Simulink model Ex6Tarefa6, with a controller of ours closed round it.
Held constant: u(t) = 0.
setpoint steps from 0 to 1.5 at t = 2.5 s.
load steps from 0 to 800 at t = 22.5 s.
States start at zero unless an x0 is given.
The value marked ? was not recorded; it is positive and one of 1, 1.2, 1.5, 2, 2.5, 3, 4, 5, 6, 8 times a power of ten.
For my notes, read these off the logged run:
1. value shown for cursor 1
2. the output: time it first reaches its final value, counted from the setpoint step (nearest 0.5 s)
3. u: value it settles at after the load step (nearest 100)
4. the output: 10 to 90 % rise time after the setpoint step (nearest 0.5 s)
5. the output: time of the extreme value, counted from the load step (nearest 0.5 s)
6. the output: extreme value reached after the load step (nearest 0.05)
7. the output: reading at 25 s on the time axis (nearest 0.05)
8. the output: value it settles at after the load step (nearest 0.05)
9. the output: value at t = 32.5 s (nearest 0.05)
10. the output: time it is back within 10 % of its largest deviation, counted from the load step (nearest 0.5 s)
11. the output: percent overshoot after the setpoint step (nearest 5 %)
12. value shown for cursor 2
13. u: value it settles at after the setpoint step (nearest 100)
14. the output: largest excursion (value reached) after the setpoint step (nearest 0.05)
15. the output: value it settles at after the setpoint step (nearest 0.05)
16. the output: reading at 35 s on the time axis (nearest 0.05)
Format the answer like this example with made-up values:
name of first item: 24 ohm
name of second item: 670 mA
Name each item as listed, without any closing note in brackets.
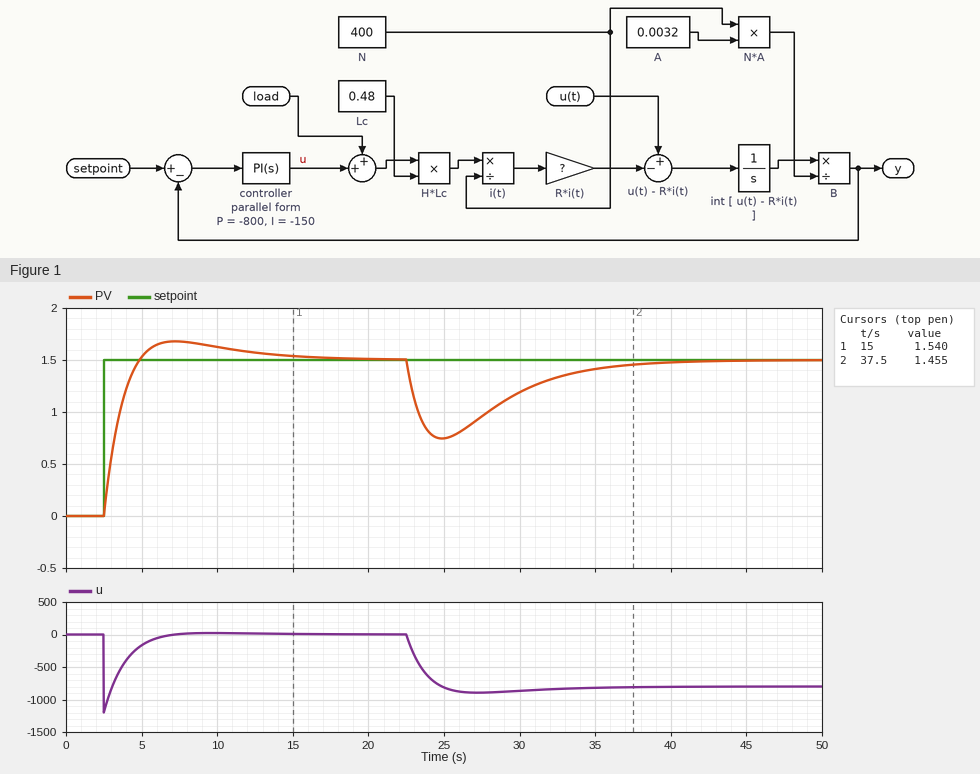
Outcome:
value shown for cursor 1: 1.540
the output: time it first reaches its final value, counted from the setpoint step: 2.5 s
u: value it settles at after the load step: -800
the output: 10 to 90 % rise time after the setpoint step: 1.5 s
the output: time of the extreme value, counted from the load step: 2.5 s
the output: extreme value reached after the load step: 0.75
the output: reading at 25 s on the time axis: 0.75
the output: value it settles at after the load step: 1.50
the output: value at t = 32.5 s: 1.35
the output: time it is back within 10 % of its largest deviation, counted from the load step: 13.0 s
the output: percent overshoot after the setpoint step: 10 %
value shown for cursor 2: 1.455
u: value it settles at after the setpoint step: 0
the output: largest excursion (value reached) after the setpoint step: 1.70
the output: value it settles at after the setpoint step: 1.50
the output: reading at 35 s on the time axis: 1.40
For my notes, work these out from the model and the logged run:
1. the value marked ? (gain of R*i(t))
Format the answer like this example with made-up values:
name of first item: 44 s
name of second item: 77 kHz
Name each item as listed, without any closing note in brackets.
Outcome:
the value marked ? (gain of R*i(t)): 1.2
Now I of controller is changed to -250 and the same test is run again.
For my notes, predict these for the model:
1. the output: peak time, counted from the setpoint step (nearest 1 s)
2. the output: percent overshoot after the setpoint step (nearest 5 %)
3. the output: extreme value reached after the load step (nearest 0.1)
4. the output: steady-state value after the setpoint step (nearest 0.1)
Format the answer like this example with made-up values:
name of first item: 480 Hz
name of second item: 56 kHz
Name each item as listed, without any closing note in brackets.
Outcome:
the output: peak time, counted from the setpoint step: 4 s
the output: percent overshoot after the setpoint step: 15 %
the output: extreme value reached after the load step: 0.8
the output: steady-state value after the setpoint step: 1.5
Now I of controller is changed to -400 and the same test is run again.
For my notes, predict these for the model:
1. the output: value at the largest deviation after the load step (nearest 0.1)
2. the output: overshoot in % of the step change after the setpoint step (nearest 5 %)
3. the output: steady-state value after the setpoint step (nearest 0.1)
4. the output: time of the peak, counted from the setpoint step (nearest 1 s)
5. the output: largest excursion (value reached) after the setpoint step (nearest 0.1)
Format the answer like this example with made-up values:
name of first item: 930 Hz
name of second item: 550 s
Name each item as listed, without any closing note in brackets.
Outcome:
the output: value at the largest deviation after the load step: 0.9
the output: overshoot in % of the step change after the setpoint step: 20 %
the output: steady-state value after the setpoint step: 1.5
the output: time of the peak, counted from the setpoint step: 3 s
the output: largest excursion (value reached) after the setpoint step: 1.8
